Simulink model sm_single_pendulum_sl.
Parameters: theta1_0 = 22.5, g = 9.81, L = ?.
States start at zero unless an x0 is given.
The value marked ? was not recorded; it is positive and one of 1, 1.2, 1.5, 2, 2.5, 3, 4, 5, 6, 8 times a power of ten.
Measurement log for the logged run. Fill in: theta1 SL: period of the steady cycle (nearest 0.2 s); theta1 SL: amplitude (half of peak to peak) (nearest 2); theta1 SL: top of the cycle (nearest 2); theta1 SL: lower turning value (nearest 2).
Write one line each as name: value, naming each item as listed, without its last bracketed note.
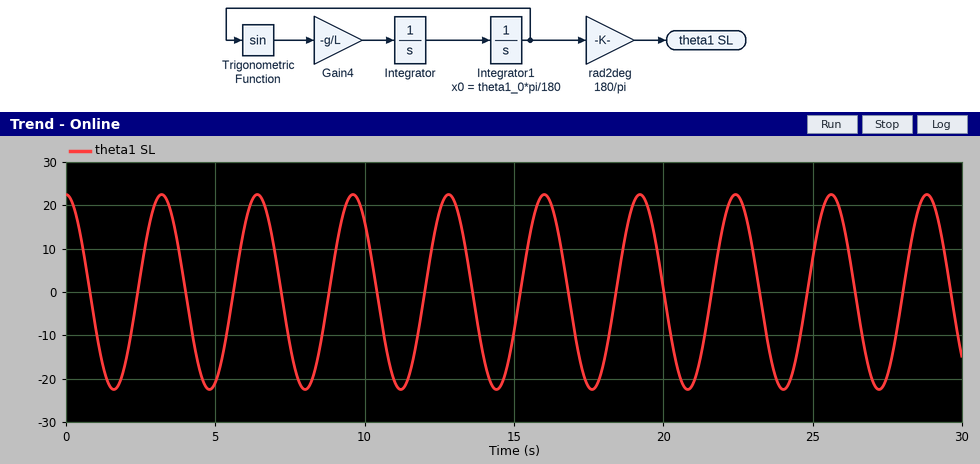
theta1 SL: period of the steady cycle: 3.2 s
theta1 SL: amplitude (half of peak to peak): 22
theta1 SL: top of the cycle: 22
theta1 SL: lower turning value: -22
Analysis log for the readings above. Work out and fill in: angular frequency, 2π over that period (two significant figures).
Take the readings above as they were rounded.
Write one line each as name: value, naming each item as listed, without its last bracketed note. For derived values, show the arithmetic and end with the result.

angular frequency, 2π over that period: 2π / 3.2 = 2.0 rad/s
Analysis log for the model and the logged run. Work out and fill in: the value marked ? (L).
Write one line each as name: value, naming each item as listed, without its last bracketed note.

the value marked ?: 2.5
